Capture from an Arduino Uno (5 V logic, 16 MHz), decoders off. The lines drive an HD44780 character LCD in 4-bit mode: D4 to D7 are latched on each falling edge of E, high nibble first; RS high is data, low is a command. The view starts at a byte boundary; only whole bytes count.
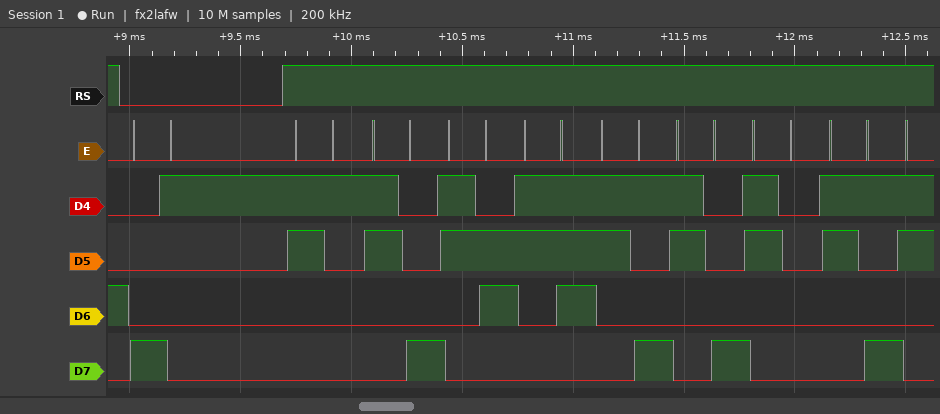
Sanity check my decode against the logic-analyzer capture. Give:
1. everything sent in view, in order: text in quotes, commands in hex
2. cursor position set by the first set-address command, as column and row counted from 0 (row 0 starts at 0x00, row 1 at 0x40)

0x81 "18679809"
column 1, row 0
